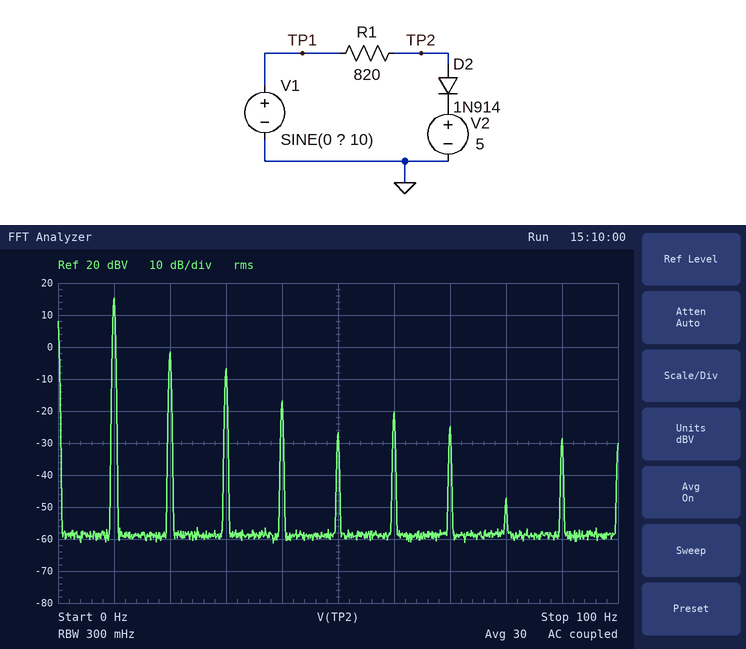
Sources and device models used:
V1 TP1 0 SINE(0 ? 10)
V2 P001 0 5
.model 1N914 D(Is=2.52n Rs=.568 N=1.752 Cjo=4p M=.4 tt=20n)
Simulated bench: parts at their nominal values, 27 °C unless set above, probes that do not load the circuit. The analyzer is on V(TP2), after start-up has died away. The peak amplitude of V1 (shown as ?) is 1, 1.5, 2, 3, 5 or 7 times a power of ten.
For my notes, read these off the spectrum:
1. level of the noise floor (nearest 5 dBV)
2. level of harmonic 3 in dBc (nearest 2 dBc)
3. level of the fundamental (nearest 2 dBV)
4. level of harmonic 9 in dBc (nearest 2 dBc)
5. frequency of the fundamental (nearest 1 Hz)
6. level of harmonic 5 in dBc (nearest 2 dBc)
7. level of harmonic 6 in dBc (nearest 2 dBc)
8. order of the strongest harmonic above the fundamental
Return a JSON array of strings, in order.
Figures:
["-60 dBV", "-22 dBc", "16 dBV", "-44 dBc", "10 Hz", "-42 dBc", "-36 dBc", "2"]
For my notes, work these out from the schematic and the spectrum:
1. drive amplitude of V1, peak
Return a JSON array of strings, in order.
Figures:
["10 V"]
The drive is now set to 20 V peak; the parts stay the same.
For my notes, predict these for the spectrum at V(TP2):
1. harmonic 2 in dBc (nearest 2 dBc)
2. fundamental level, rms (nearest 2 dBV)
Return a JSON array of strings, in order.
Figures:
["-12 dBc", "20 dBV"]
